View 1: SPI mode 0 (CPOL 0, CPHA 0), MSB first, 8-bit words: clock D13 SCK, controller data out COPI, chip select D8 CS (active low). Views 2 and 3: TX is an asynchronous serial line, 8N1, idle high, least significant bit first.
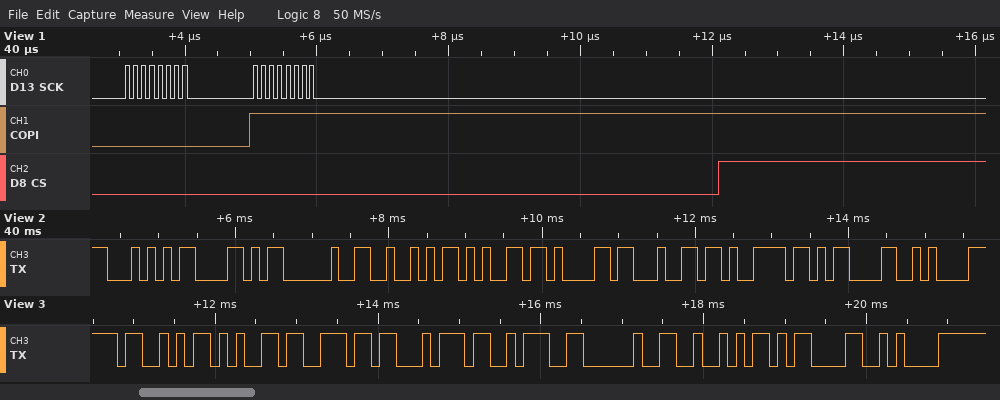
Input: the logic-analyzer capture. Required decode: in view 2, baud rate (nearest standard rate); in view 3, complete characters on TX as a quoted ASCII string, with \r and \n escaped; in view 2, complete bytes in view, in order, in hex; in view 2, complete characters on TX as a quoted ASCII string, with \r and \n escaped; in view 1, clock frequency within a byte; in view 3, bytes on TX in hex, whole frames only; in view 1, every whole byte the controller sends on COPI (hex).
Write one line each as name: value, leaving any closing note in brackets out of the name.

in view 2, baud rate: 9600 baud
in view 3, complete characters on TX as a quoted ASCII string, with \r and \n escaped: "Sent: R\r\n"
in view 2, complete bytes in view, in order, in hex: 0x54 0x58 0x20 0x52 0x65 0x61 0x64 0x79 0x0D 0x0A
in view 2, complete characters on TX as a quoted ASCII string, with \r and \n escaped: "TX Ready\r\n"
in view 1, clock frequency within a byte: 8 MHz
in view 3, bytes on TX in hex, whole frames only: 53 65 6E 74 3A 20 52 0D 0A
in view 1, every whole byte the controller sends on COPI: 0x00 0xFF
